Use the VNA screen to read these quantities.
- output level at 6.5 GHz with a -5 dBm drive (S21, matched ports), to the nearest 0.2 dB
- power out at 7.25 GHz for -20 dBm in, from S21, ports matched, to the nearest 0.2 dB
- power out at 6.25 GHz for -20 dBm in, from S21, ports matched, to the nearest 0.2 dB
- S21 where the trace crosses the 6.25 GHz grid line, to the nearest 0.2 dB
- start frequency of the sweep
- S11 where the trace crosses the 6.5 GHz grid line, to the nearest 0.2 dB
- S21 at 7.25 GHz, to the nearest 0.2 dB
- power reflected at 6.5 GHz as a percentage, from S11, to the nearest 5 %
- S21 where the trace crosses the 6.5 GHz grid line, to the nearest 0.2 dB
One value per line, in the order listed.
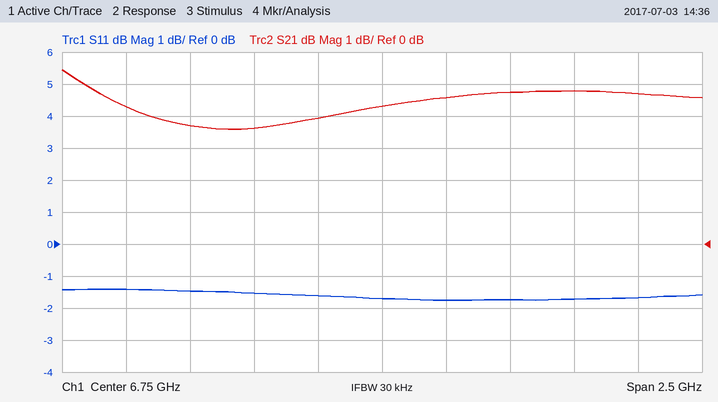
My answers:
-1.0 dBm
-15.2 dBm
-16.4 dBm
3.6 dB
5.5 GHz
-1.6 dB
4.8 dB
70 %
4.0 dB
